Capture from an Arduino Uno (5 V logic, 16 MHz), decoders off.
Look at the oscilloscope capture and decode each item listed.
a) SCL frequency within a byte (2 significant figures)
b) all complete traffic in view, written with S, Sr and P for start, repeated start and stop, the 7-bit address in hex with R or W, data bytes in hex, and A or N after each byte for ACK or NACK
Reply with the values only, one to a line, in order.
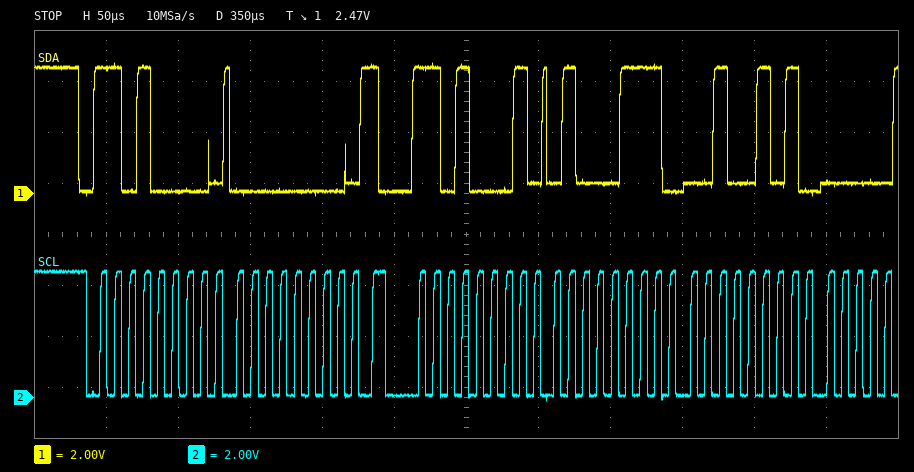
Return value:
100 kHz
S 68W A 00 A Sr 68R A 47 A 25 A
